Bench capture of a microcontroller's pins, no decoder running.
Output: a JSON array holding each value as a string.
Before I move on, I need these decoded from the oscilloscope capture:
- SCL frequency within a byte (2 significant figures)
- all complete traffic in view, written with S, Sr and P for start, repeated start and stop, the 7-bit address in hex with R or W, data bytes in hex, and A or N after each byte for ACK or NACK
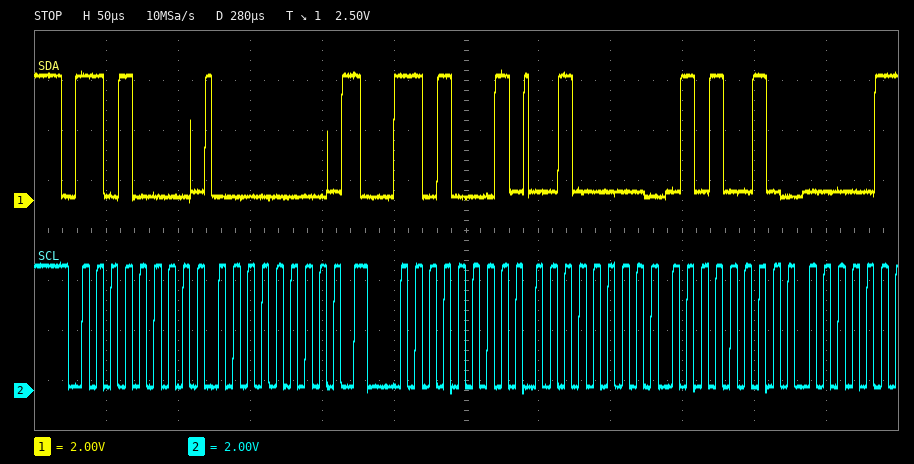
["100 kHz", "S 68W A 00 A Sr 68R A 20 A 52 A"]
